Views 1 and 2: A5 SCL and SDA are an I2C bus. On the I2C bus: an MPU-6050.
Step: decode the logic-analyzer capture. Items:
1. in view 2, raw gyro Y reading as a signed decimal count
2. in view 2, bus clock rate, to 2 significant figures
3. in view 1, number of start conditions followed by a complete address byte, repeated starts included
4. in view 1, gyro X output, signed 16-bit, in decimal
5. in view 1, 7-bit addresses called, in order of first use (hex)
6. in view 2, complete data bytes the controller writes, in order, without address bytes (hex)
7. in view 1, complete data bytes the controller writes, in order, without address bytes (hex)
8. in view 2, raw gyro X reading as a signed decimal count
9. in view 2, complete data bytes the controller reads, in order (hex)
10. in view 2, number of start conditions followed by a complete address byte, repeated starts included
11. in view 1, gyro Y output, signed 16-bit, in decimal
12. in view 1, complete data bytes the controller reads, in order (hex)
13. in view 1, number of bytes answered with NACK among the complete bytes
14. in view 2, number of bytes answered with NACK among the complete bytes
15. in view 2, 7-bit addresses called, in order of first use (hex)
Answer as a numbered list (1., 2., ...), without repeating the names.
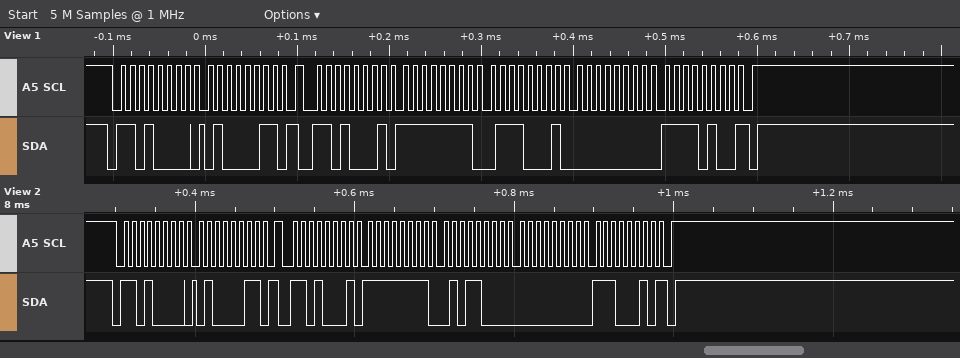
1. 226
2. 100 kHz
3. 2
4. -143
5. 0x68
6. 43
7. 43
8. -168
9. FF 58 00 E2
10. 2
11. 244
12. FF 71 00 F4
13. 1
14. 1
15. 0x68
